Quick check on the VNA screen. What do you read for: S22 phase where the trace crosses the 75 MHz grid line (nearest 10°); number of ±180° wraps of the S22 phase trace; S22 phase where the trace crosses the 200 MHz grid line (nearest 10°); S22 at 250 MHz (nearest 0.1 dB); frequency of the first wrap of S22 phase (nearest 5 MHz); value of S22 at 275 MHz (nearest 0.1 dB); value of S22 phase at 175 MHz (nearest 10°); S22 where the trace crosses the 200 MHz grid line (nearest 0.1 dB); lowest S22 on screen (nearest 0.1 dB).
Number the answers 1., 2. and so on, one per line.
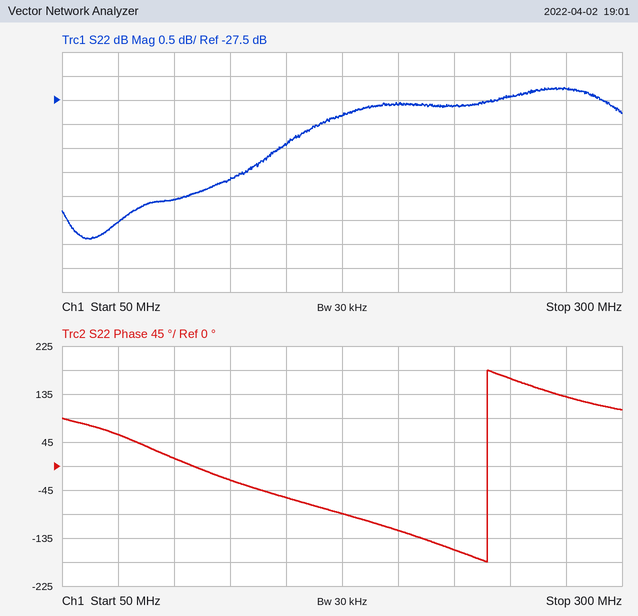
1. 60°
2. 1
3. -120°
4. -27.4 dB
5. 240 MHz
6. -27.3 dB
7. -90°
8. -27.6 dB
9. -30.4 dB
